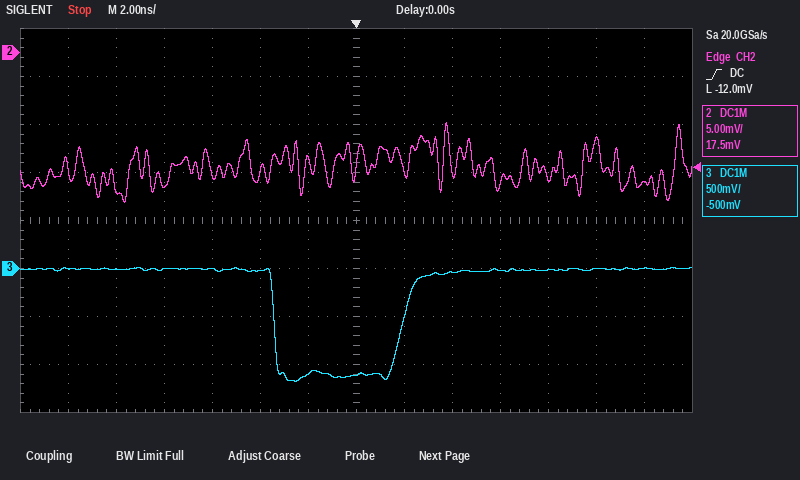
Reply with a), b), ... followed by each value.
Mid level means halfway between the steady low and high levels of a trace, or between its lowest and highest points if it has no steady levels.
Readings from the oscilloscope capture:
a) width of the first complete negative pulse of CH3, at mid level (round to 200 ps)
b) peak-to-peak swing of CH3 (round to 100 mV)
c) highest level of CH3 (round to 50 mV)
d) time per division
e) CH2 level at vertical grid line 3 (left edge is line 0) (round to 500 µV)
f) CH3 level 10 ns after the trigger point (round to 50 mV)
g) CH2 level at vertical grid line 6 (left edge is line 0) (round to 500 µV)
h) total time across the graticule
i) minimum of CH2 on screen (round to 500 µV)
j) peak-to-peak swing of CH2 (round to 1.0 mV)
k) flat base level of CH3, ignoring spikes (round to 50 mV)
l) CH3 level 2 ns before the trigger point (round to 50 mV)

a) 5.4 ns
b) 1.20 V
c) 0 mV
d) 2 ns
e) -14.0 mV
f) 0 mV
g) -11.0 mV
h) 28 ns
i) -15.5 mV
j) 8.0 mV
k) -1.10 V
l) -1.10 V
